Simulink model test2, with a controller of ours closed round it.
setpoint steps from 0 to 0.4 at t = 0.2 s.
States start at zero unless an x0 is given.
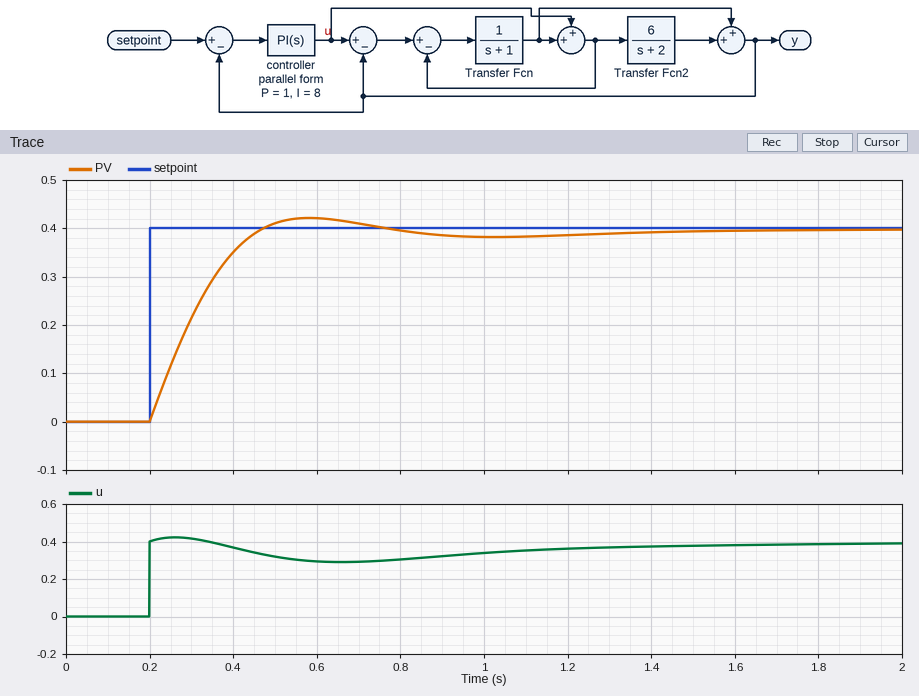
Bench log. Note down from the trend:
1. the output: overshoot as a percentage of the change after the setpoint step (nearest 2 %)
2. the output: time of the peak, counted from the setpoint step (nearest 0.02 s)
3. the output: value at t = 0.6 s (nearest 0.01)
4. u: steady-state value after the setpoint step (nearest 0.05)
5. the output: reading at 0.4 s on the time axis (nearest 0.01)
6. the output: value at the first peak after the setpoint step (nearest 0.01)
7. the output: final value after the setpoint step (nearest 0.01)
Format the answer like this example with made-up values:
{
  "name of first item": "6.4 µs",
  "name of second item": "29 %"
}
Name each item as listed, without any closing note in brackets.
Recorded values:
{
  "the output: overshoot as a percentage of the change after the setpoint step": "6 %",
  "the output: time of the peak, counted from the setpoint step": "0.38 s",
  "the output: value at t = 0.6 s": "0.42",
  "u: steady-state value after the setpoint step": "0.40",
  "the output: reading at 0.4 s on the time axis": "0.35",
  "the output: value at the first peak after the setpoint step": "0.42",
  "the output: final value after the setpoint step": "0.40"
}
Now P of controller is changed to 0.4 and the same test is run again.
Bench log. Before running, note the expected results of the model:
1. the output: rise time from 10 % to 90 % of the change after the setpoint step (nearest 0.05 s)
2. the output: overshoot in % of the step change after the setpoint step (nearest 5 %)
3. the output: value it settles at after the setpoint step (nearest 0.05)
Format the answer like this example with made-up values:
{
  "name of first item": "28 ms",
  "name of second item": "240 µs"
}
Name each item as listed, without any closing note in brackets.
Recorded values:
{
  "the output: rise time from 10 % to 90 % of the change after the setpoint step": "0.20 s",
  "the output: overshoot in % of the step change after the setpoint step": "20 %",
  "the output: value it settles at after the setpoint step": "0.40"
}
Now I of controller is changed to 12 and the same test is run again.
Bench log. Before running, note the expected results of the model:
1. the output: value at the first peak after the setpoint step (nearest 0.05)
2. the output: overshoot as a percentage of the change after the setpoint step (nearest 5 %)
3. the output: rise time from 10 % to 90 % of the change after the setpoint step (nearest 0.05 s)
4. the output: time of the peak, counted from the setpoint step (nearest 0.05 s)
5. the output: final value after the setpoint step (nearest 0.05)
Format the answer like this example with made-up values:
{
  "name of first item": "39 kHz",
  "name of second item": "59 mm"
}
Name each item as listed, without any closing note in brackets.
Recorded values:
{
  "the output: value at the first peak after the setpoint step": "0.45",
  "the output: overshoot as a percentage of the change after the setpoint step": "15 %",
  "the output: rise time from 10 % to 90 % of the change after the setpoint step": "0.15 s",
  "the output: time of the peak, counted from the setpoint step": "0.30 s",
  "the output: final value after the setpoint step": "0.40"
}
